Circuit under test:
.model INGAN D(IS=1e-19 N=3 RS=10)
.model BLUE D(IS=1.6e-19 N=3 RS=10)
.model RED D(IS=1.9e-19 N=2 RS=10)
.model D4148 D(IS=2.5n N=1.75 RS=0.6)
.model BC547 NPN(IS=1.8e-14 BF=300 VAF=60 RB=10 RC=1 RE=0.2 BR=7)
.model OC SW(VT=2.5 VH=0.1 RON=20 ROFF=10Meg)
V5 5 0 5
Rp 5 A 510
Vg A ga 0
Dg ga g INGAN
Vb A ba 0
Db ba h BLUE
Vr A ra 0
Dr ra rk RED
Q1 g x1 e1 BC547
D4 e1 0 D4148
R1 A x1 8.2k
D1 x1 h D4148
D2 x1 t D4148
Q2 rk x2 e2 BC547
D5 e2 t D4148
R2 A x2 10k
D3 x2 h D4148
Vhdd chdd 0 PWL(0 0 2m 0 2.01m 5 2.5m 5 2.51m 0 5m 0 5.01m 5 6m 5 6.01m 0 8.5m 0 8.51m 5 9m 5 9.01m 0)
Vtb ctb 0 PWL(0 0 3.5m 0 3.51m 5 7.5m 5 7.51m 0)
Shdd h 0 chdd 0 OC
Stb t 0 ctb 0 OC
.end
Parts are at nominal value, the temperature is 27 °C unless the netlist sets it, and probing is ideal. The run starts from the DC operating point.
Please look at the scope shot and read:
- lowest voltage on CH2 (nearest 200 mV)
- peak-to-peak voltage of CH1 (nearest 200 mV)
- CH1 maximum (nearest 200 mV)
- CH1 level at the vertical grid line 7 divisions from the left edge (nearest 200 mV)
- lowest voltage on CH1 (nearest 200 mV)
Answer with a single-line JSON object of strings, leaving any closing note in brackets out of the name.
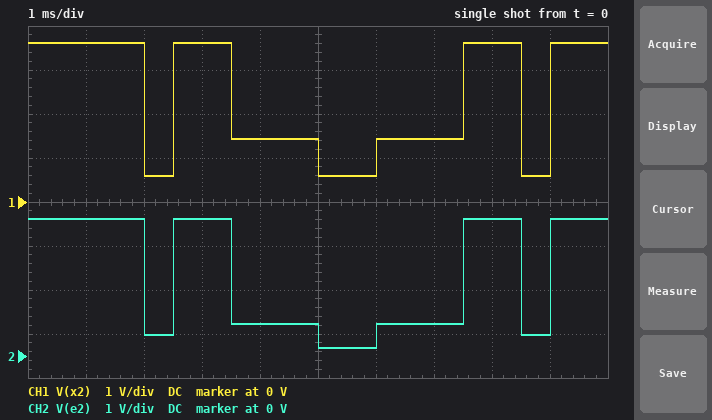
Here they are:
{"lowest voltage on CH2": "200 mV", "peak-to-peak voltage of CH1": "3.0 V", "CH1 maximum": "3.6 V", "CH1 level at the vertical grid line 7 divisions from the left edge": "1.4 V", "lowest voltage on CH1": "600 mV"}
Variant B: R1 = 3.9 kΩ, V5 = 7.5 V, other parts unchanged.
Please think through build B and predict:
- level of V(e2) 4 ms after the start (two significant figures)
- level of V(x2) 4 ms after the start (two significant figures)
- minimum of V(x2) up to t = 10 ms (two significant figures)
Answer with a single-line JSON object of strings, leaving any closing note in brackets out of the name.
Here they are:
{"level of V(e2) 4 ms after the start": "860 mV", "level of V(x2) 4 ms after the start": "1.6 V", "minimum of V(x2) up to t = 10 ms": "680 mV"}
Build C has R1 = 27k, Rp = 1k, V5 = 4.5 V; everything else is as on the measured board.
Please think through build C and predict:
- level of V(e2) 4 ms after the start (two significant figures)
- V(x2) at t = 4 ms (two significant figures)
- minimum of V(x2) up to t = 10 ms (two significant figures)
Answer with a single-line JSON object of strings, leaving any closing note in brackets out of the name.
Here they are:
{"level of V(e2) 4 ms after the start": "650 mV", "V(x2) at t = 4 ms": "1.3 V", "minimum of V(x2) up to t = 10 ms": "550 mV"}
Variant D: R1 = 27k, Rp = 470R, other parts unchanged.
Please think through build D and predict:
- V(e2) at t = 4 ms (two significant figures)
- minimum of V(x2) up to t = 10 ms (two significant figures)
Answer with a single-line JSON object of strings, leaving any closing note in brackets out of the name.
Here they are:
{"V(e2) at t = 4 ms": "750 mV", "minimum of V(x2) up to t = 10 ms": "600 mV"}
